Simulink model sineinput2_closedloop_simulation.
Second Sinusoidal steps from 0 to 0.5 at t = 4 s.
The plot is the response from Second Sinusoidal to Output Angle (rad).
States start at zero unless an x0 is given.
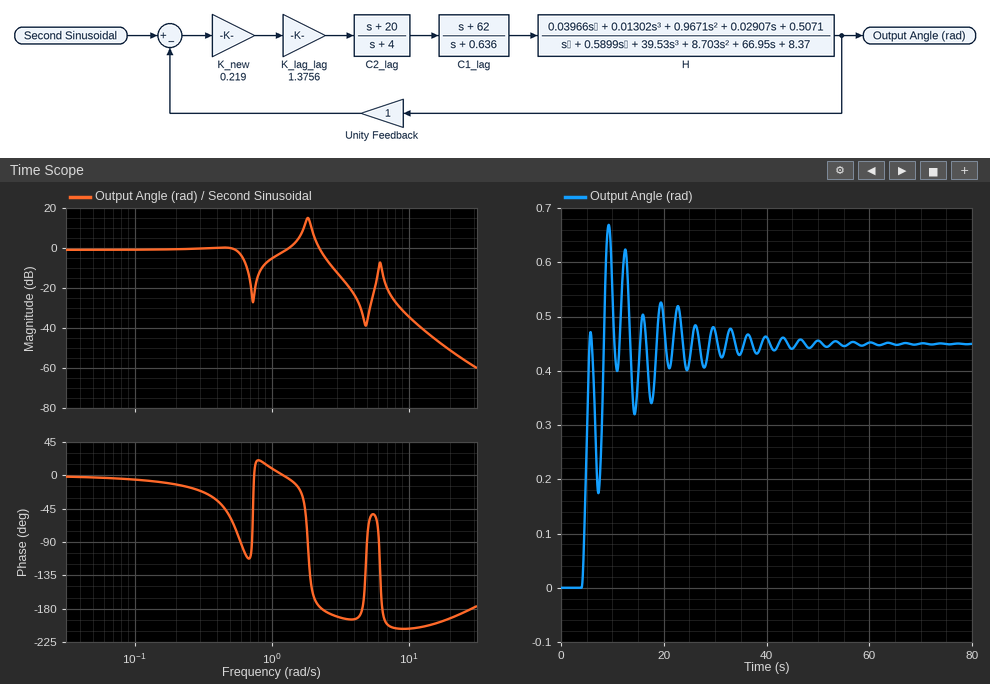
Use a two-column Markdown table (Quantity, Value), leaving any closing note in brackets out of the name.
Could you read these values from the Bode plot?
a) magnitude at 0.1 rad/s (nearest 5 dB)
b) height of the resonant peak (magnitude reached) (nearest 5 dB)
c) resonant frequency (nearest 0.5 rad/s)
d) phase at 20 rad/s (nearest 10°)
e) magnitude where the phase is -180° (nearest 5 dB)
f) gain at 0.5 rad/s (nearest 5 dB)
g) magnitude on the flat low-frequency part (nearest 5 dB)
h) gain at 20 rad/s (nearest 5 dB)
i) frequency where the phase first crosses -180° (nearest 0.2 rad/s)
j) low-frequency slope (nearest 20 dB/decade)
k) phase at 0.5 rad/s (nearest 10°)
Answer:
| Quantity | Value |
|---|---|
| magnitude at 0.1 rad/s | 0 dB |
| height of the resonant peak (magnitude reached) | 15 dB |
| resonant frequency | 2.0 rad/s |
| phase at 20 rad/s | -190° |
| magnitude where the phase is -180° | 0 dB |
| gain at 0.5 rad/s | 0 dB |
| magnitude on the flat low-frequency part | 0 dB |
| gain at 20 rad/s | -50 dB |
| frequency where the phase first crosses -180° | 2.4 rad/s |
| low-frequency slope | 0 dB/decade |
| phase at 0.5 rad/s | -60° |
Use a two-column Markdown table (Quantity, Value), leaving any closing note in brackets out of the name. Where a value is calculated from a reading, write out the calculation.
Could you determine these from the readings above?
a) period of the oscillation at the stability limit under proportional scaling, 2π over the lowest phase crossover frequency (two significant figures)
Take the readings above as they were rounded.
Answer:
| Quantity | Value |
|---|---|
| period of the oscillation at the stability limit under proportional scaling, 2π over the lowest phase crossover frequency | 2π / 2.4 = 2.6 s |
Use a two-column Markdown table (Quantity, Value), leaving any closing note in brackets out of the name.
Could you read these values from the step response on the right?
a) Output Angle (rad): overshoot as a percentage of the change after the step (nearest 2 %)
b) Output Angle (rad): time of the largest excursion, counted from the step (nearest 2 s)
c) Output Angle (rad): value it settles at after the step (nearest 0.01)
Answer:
| Quantity | Value |
|---|---|
| Output Angle (rad): overshoot as a percentage of the change after the step | 48 % |
| Output Angle (rad): time of the largest excursion, counted from the step | 6 s |
| Output Angle (rad): value it settles at after the step | 0.45 |
